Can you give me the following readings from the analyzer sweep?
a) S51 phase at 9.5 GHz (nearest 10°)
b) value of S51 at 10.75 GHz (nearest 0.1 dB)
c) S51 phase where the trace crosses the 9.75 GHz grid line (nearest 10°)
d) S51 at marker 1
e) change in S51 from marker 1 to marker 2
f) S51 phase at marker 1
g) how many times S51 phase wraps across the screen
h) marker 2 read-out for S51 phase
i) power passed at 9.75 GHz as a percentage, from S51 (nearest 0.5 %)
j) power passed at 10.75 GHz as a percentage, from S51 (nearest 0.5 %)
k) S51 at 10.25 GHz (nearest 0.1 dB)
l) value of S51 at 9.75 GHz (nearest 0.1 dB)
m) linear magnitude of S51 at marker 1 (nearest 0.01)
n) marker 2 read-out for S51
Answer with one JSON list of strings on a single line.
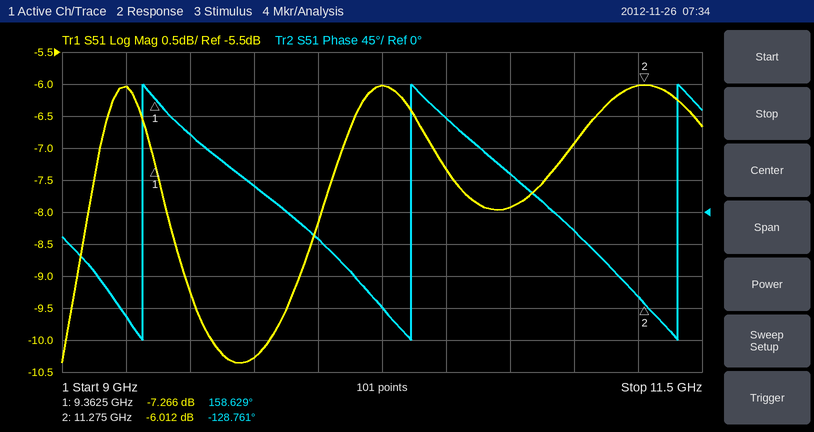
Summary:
["110°", "-7.9 dB", "40°", "-7.266 dB", "1.254 dB", "158.629°", "3", "-128.761°", "9.5 %", "16.0 %", "-6.0 dB", "-10.3 dB", "0.43", "-6.012 dB"]
